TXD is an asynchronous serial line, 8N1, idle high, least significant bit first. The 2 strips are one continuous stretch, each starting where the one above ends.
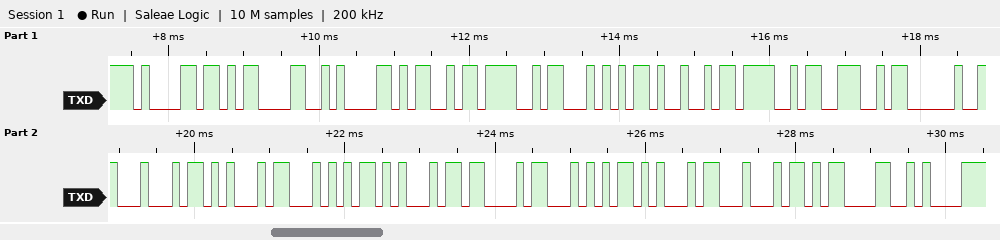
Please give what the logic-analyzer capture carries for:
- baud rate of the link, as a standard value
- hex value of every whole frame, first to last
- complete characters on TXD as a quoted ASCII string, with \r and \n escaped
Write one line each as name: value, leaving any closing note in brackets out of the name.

baud rate of the link, as a standard value: 9600 baud
hex value of every whole frame, first to last: 61 0D 0A 4D 4F 54 49 4F 4E 20 44 45 54 45 43 54 45 44 0D 0A
complete characters on TXD as a quoted ASCII string, with \r and \n escaped: "a\r\nMOTION DETECTED\r\n"
